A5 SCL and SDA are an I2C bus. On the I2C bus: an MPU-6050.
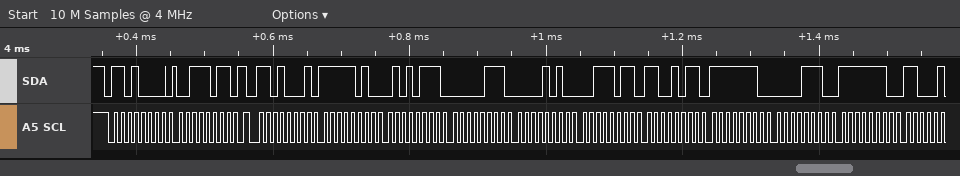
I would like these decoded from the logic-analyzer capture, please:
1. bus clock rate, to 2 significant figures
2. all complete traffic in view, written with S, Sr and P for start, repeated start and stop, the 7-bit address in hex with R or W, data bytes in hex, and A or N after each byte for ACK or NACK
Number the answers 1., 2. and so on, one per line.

1. 100 kHz
2. S 68W A 3B A Sr 68R A FA A 57 A 07 A 0A A 3B A CB A FE A 0E A FE A
